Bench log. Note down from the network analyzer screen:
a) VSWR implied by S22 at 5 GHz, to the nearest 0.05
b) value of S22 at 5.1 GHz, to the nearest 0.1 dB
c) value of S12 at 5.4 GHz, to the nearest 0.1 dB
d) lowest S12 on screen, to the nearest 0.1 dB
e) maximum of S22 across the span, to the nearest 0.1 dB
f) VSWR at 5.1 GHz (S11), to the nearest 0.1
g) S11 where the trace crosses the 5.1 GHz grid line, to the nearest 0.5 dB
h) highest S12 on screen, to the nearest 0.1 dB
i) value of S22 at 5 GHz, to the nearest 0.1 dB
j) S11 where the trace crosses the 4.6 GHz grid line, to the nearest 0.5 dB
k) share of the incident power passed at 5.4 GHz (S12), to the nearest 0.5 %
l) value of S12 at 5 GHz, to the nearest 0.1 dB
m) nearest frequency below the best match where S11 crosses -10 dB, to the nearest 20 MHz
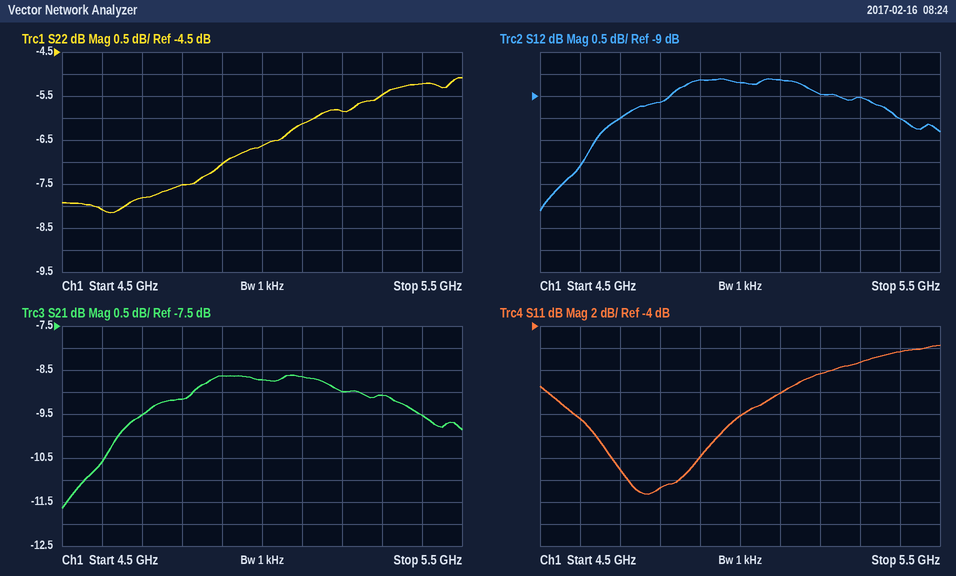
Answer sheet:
2.75
-6.1 dB
-9.5 dB
-11.6 dB
-5.1 dB
1.9
-10.0 dB
-8.6 dB
-6.6 dB
-12.5 dB
11.0 %
-8.7 dB
4.52 GHz
